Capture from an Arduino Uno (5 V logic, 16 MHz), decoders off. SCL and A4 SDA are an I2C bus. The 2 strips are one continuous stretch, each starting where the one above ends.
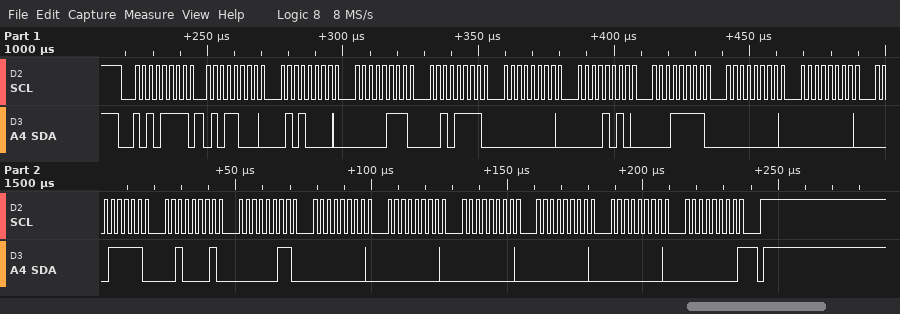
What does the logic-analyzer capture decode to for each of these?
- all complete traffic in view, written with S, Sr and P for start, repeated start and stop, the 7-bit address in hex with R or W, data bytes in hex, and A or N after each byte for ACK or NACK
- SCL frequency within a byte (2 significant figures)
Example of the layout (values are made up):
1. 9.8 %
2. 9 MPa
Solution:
1. S 57R A 58 A 50 A 07 A 2F A 00 A 0A A 1F A 00 A 00 A 1F A 21 A 03 A 00 A 00 A 00 A 00 A 00 A 00 N P
2. 400 kHz
